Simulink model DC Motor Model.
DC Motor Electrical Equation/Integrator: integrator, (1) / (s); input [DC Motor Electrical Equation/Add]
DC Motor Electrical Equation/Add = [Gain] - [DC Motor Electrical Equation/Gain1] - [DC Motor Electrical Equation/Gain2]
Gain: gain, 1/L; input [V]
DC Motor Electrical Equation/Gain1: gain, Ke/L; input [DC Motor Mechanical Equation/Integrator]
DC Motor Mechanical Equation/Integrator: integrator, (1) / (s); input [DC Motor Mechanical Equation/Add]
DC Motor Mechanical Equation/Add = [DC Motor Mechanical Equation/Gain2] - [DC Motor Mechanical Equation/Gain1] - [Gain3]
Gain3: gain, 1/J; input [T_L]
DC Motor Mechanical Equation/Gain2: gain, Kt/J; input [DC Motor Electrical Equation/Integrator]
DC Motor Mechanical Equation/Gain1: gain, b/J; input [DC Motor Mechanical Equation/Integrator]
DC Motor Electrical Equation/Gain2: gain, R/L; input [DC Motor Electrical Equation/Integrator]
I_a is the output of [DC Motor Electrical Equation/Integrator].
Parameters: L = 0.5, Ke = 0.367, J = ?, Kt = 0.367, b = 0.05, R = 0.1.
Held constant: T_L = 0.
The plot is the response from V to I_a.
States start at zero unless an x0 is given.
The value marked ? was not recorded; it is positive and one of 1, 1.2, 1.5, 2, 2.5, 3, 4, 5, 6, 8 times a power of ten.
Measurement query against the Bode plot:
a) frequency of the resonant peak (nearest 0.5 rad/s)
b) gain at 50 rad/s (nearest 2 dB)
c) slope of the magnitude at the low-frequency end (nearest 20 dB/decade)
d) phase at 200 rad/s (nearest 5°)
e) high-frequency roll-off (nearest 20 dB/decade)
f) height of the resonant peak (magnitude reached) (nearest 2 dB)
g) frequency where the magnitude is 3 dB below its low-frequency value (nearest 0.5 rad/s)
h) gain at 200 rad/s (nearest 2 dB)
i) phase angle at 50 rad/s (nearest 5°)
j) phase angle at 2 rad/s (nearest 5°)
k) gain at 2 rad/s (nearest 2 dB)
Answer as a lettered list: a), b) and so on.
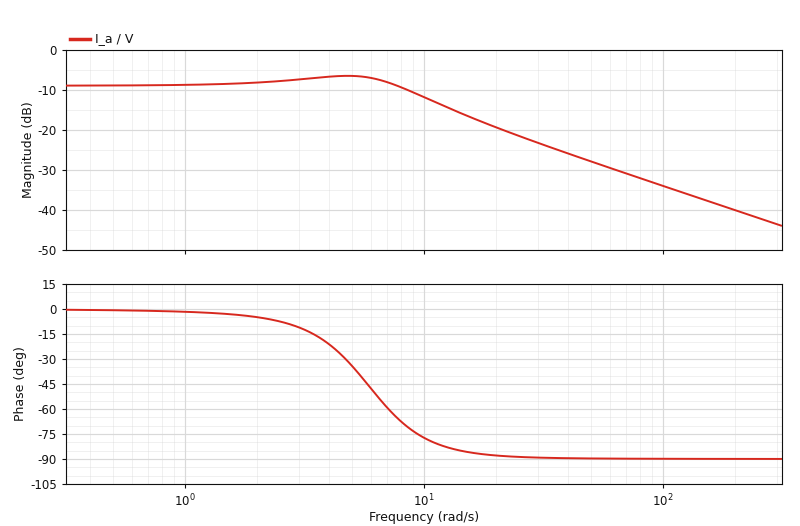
a) 4.5 rad/s
b) -28 dB
c) 0 dB/decade
d) -90°
e) -20 dB/decade
f) -6 dB
g) 10.0 rad/s
h) -40 dB
i) -90°
j) -5°
k) -8 dB
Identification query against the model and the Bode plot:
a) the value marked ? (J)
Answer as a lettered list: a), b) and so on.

a) 0.008
